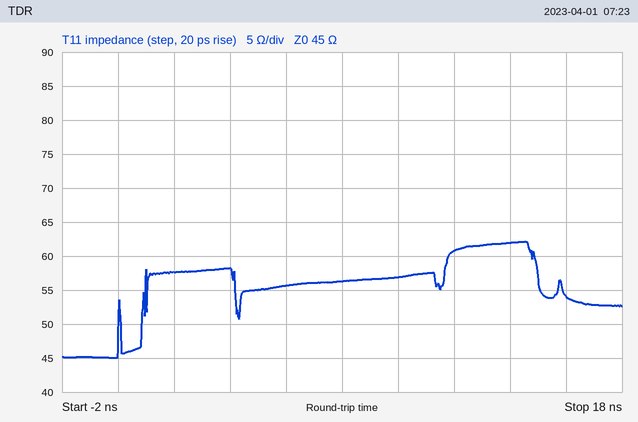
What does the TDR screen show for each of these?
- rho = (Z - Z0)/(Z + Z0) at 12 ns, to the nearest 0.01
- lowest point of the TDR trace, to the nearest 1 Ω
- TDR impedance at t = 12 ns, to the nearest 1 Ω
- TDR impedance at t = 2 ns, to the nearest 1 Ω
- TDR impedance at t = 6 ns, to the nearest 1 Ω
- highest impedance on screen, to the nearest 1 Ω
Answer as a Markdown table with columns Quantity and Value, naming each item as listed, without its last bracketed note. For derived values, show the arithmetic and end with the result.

| Quantity | Value |
|---|---|
| rho = (Z - Z0)/(Z + Z0) at 12 ns, to the nearest 0.01 | (61 − 45)/(61 + 45) ≈ +0.15 |
| lowest point of the TDR trace, to the nearest 1 Ω | 45 Ω |
| TDR impedance at t = 12 ns, to the nearest 1 Ω | 61 Ω |
| TDR impedance at t = 2 ns, to the nearest 1 Ω | 58 Ω |
| TDR impedance at t = 6 ns, to the nearest 1 Ω | 56 Ω |
| highest impedance on screen, to the nearest 1 Ω | 62 Ω |
